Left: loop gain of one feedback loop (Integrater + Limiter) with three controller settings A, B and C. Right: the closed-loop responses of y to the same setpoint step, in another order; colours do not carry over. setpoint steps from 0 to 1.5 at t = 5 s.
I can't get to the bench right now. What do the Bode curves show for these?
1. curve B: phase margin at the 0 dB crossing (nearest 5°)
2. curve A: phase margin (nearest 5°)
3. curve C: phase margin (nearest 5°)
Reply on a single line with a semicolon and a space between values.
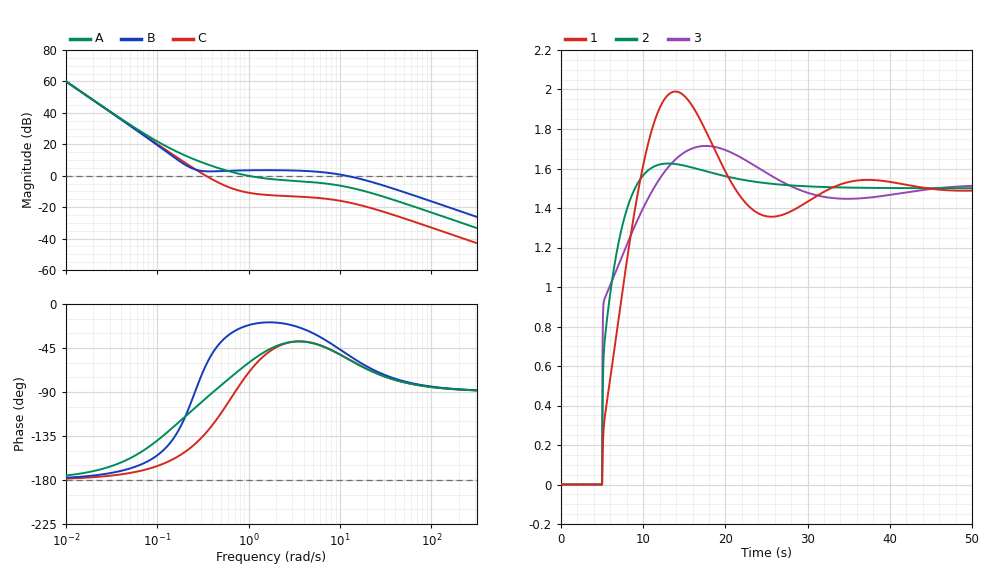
130°; 120°; 50°
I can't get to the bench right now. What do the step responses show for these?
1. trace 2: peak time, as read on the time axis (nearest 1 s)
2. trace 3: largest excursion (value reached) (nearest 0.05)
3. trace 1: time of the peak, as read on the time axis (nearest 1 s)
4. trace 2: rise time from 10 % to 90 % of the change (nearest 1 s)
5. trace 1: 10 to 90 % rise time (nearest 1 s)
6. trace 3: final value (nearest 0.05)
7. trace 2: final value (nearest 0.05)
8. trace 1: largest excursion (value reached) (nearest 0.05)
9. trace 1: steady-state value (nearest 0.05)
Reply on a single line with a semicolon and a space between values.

13 s; 1.70; 14 s; 3 s; 4 s; 1.50; 1.50; 2.00; 1.50
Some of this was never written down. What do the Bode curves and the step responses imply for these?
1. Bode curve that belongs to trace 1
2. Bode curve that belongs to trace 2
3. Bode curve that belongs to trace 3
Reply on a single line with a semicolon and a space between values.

C; A; B
